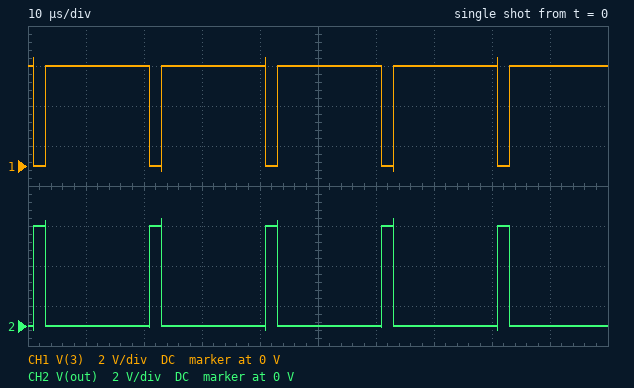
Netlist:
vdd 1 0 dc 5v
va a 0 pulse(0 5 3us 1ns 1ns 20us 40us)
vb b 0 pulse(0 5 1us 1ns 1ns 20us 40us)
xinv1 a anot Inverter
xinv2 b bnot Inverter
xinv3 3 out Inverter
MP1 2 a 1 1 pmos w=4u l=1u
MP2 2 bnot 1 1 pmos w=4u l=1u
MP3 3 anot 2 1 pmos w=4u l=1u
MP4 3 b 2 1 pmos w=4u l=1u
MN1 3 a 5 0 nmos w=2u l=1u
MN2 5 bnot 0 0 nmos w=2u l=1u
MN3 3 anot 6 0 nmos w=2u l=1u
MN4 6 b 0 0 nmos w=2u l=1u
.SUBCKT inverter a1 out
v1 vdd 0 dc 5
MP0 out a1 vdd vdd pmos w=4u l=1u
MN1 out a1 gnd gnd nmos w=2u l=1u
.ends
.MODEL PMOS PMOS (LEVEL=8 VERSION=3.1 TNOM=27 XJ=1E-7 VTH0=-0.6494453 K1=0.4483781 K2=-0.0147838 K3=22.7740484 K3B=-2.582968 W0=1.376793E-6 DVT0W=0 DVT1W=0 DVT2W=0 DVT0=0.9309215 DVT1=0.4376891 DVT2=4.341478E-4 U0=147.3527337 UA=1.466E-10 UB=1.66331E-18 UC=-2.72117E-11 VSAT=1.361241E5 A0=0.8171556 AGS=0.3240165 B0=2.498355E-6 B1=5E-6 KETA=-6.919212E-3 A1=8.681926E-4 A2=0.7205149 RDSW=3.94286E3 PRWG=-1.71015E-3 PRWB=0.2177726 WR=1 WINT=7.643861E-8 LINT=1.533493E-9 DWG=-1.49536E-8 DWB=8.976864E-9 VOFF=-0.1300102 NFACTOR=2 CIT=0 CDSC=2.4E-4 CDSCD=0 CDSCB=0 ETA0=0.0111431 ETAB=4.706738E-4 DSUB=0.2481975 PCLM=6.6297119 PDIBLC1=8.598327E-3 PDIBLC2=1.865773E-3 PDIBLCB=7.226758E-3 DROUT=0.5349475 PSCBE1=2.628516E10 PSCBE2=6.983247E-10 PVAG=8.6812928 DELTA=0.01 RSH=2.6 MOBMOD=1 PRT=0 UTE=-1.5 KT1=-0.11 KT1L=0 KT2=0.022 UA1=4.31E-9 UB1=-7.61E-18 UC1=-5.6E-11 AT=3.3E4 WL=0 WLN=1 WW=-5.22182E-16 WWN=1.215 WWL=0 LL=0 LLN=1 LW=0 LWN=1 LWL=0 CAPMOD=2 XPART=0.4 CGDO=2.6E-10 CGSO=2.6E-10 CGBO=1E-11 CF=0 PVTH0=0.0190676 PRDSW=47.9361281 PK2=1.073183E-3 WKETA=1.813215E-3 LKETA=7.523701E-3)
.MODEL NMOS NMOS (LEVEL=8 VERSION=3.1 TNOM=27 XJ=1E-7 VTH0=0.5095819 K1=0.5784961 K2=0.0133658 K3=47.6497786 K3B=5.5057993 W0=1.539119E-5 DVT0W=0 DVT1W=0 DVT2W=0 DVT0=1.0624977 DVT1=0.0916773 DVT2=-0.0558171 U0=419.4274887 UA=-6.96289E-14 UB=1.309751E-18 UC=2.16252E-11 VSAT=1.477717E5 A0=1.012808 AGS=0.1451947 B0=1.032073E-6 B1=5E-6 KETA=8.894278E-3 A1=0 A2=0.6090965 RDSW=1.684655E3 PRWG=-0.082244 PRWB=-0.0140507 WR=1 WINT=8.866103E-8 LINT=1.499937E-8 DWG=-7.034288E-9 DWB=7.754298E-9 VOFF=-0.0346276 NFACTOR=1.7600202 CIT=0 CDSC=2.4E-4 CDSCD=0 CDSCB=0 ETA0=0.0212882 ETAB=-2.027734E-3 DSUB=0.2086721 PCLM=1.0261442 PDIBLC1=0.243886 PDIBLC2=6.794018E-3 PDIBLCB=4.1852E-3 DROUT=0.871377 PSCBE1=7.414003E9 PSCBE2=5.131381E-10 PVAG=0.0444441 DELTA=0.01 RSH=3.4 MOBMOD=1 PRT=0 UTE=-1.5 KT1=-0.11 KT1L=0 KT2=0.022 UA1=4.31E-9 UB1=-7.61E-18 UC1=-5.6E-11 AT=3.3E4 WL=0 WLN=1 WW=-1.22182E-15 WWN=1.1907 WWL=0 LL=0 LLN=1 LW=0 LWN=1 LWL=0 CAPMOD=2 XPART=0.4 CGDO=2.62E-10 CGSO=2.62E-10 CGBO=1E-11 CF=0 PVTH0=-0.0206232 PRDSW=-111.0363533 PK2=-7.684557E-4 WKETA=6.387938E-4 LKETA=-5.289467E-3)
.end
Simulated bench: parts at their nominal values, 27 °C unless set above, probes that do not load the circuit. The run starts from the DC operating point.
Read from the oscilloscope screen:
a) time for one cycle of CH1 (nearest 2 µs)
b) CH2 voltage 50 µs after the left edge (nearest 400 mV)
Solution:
20 µs
0 V
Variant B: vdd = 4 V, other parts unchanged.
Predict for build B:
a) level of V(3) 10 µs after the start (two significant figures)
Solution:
4.0 V
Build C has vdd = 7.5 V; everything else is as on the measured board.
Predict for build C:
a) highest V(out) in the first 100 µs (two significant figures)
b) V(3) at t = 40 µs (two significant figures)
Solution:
4.4 V
7.5 V
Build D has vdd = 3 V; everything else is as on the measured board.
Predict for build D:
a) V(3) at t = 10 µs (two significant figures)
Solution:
3.0 V
